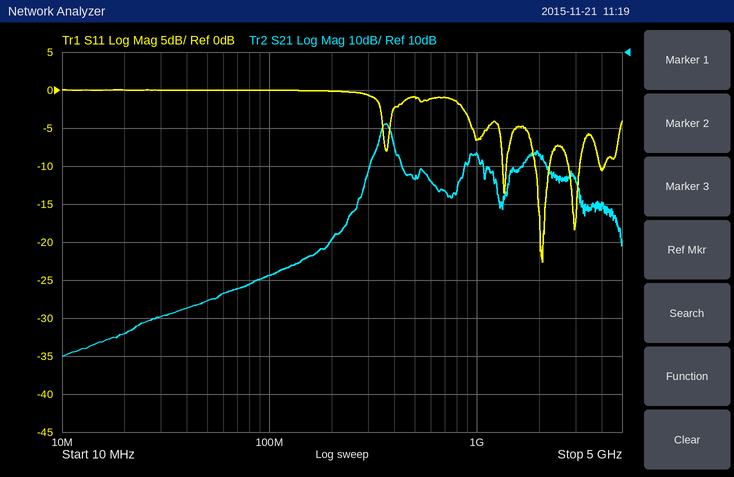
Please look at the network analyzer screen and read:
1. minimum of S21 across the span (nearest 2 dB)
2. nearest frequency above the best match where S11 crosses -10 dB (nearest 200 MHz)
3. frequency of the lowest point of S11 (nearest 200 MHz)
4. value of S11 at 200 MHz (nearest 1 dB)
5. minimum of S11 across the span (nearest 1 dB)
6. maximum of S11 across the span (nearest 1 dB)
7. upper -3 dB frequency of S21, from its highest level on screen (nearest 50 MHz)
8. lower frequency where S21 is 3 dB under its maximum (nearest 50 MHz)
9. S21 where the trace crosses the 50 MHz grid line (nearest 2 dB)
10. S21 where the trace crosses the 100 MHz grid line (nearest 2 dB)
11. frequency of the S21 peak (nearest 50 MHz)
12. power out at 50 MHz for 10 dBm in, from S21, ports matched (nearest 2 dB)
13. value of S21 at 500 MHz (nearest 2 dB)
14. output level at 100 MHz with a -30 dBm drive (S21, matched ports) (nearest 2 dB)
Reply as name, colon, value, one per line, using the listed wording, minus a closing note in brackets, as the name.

minimum of S21 across the span: -70 dB
nearest frequency above the best match where S11 crosses -10 dB: 2.2 GHz
frequency of the lowest point of S11: 2.0 GHz
value of S11 at 200 MHz: 0 dB
minimum of S11 across the span: -23 dB
maximum of S11 across the span: 0 dB
upper -3 dB frequency of S21, from its highest level on screen: 400 MHz
lower frequency where S21 is 3 dB under its maximum: 350 MHz
S21 where the trace crosses the 50 MHz grid line: -56 dB
S21 where the trace crosses the 100 MHz grid line: -48 dB
frequency of the S21 peak: 350 MHz
power out at 50 MHz for 10 dBm in, from S21, ports matched: -46 dBm
value of S21 at 500 MHz: -24 dB
output level at 100 MHz with a -30 dBm drive (S21, matched ports): -78 dBm
